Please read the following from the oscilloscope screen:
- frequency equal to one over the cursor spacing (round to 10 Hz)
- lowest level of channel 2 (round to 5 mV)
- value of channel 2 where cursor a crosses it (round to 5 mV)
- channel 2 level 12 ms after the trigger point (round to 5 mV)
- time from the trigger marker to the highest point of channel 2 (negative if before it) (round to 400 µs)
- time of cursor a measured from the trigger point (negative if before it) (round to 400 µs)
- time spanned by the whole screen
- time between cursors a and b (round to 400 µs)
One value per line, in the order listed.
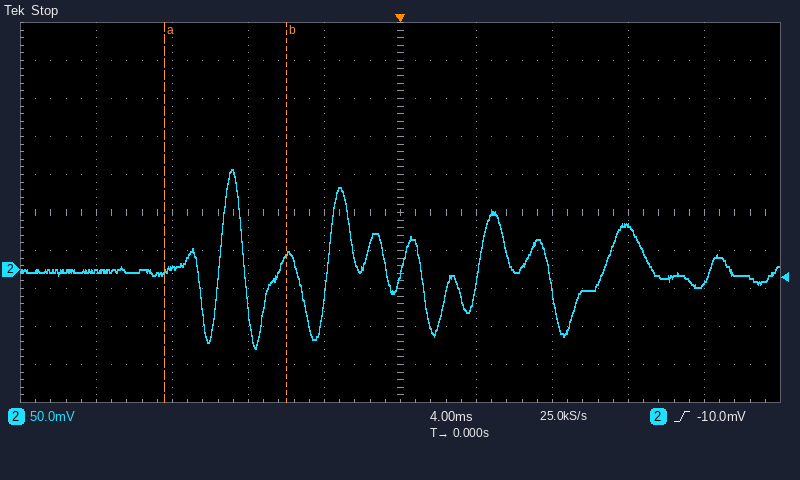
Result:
160 Hz
-105 mV
-5 mV
55 mV
-8.8 ms
-12.4 ms
40 ms
6.4 ms
